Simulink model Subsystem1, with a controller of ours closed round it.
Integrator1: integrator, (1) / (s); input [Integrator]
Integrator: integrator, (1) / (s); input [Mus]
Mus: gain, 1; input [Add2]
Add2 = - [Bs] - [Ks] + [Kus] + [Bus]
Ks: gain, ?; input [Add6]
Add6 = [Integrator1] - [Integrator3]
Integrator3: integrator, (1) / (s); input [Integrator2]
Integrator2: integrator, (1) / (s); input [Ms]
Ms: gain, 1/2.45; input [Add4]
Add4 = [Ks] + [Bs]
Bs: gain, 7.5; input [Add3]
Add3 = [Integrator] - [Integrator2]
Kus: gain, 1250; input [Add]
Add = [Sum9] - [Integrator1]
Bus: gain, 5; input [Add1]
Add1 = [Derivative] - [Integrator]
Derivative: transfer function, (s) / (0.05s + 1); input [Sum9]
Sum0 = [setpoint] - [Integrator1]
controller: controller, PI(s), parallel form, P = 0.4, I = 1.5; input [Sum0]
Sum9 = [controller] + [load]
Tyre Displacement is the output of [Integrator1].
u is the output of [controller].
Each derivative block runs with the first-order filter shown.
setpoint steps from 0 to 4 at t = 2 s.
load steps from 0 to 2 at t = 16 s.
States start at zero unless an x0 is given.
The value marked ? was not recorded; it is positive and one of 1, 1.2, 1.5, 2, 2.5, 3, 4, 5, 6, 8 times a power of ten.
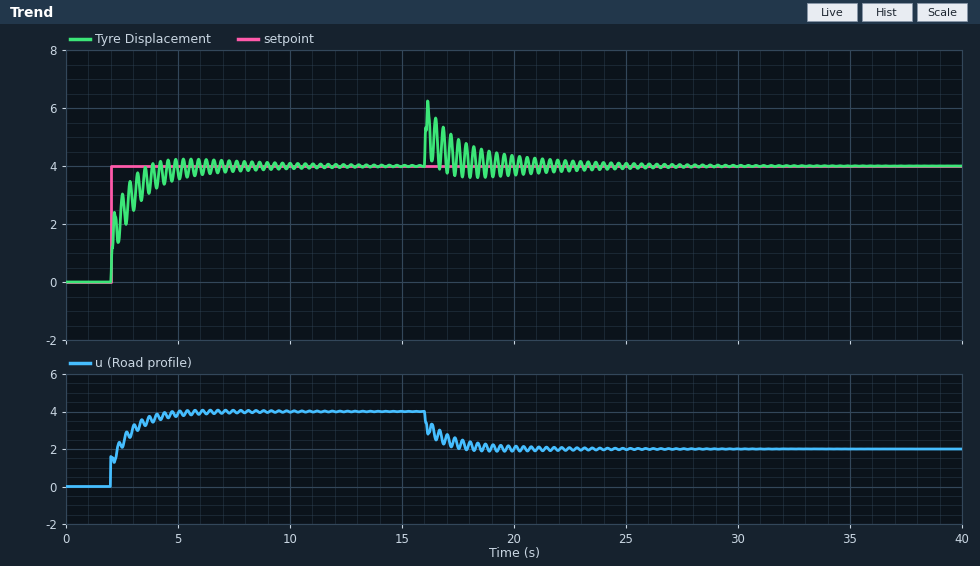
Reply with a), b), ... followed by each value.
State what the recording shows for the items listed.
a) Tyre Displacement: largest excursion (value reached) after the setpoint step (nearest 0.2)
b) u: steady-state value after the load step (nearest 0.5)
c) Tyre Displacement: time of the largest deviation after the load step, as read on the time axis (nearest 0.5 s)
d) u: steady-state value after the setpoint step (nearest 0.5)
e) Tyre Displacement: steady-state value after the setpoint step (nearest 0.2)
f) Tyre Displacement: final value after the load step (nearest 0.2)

a) 4.2
b) 2.0
c) 16.0 s
d) 4.0
e) 4.0
f) 4.0
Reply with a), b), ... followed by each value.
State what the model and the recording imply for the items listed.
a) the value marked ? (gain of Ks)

a) 2000
